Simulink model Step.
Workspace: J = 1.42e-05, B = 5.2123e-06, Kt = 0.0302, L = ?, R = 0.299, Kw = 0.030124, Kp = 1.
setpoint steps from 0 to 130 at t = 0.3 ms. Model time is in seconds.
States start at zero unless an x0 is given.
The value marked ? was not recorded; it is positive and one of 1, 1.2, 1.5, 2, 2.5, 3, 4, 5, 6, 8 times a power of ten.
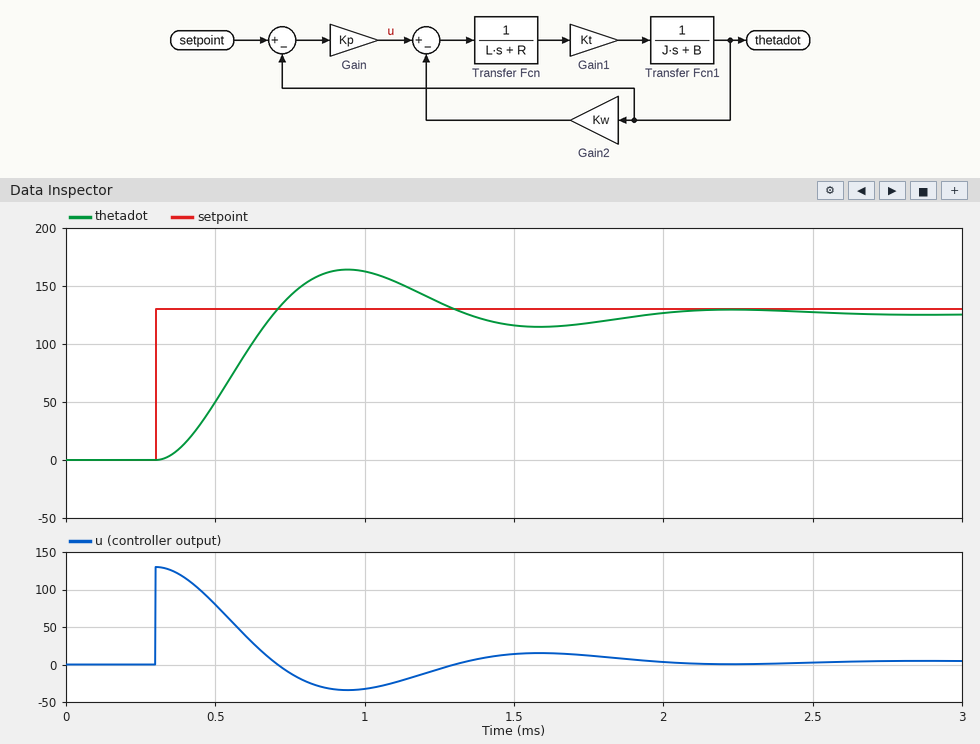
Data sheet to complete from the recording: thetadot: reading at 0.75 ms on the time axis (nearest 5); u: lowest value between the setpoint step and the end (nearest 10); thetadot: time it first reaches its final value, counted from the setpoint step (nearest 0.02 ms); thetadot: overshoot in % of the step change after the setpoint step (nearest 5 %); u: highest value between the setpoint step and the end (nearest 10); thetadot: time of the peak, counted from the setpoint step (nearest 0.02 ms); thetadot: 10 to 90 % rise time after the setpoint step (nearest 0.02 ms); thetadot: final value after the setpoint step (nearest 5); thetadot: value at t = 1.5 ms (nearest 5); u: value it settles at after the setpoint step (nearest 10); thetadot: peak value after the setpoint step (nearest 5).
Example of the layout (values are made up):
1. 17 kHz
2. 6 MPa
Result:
1. 140
2. -30
3. 0.40 ms
4. 30 %
5. 130
6. 0.64 ms
7. 0.26 ms
8. 125
9. 115
10. 0
11. 165
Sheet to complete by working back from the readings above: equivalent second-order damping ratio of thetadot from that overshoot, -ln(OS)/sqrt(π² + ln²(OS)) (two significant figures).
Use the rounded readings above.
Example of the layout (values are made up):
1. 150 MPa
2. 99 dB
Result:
1. 0.36
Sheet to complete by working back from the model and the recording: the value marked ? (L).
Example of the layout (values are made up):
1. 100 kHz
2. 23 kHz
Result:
1. 8e-05
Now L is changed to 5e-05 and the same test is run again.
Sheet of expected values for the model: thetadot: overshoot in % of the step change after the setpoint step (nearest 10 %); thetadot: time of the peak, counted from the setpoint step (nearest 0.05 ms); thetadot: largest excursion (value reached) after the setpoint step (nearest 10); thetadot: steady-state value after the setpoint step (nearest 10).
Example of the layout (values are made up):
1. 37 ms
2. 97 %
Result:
1. 20 %
2. 0.55 ms
3. 150
4. 130
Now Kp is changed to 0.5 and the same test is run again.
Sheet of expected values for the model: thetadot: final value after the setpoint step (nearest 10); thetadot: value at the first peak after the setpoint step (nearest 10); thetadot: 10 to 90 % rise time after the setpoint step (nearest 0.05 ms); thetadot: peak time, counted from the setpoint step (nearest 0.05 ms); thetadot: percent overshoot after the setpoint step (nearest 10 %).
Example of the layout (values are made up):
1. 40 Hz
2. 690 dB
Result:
1. 120
2. 140
3. 0.45 ms
4. 0.95 ms
5. 20 %
